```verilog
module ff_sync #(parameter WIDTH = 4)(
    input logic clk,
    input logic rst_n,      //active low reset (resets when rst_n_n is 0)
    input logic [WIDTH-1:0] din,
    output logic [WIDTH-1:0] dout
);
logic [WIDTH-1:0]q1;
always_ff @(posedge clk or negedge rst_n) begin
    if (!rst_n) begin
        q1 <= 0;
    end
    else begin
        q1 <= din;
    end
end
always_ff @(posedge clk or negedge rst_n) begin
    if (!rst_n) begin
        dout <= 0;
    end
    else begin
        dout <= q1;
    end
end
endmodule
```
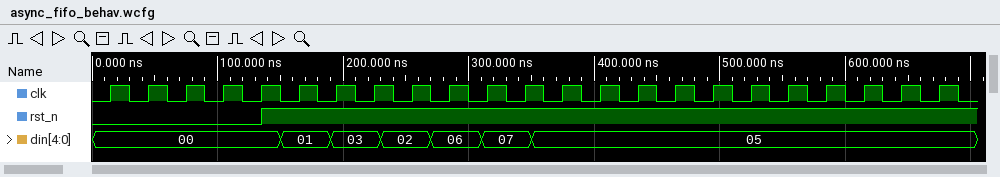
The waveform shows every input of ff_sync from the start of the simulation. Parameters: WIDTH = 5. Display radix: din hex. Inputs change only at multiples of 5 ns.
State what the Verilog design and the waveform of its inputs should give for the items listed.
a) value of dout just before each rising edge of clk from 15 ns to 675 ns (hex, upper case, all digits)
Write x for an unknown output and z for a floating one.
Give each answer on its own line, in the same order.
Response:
00, 00, 00, 00, 00, 00, 00, 01, 03, 03, 02, 06, 07, 07, 05, 05, 05, 05, 05, 05, 05, 05, 05
